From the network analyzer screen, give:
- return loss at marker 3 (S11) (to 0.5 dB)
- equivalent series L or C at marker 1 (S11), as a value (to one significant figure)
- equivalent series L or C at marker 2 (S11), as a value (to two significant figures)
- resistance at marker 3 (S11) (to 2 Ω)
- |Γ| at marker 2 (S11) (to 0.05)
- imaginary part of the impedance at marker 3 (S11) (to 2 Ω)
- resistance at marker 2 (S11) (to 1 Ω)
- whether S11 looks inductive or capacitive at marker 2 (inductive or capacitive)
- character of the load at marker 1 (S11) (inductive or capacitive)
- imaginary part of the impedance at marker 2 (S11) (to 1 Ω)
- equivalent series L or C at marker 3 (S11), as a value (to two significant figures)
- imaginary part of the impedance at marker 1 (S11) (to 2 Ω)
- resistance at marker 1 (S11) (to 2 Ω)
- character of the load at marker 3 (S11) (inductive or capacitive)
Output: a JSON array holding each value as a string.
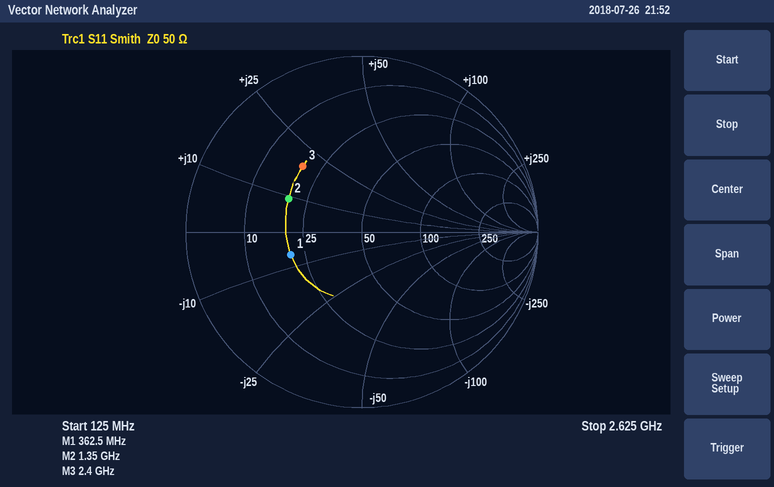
["6.0 dB", "70 pF", "1.1 nH", "20 Ω", "0.45", "+20 Ω", "19 Ω", "inductive", "capacitive", "+9 Ω", "1.3 nH", "-6 Ω", "20 Ω", "inductive"]
